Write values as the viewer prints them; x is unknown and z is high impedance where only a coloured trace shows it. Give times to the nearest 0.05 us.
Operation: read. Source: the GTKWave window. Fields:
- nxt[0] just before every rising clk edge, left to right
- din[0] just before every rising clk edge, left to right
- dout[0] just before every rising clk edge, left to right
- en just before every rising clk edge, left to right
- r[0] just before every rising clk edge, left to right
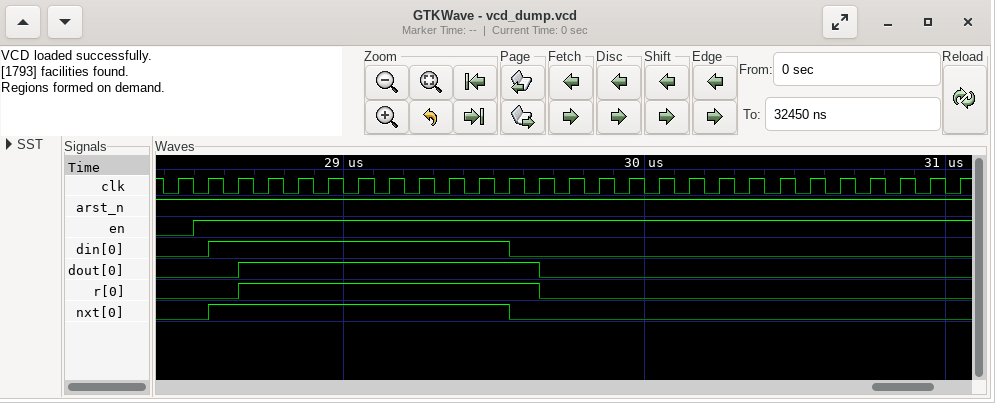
0 0 1 1 1 1 1 1 1 1 1 1 0 0 0 0 0 0 0 0 0 0 0 0 0 0 0
0 0 1 1 1 1 1 1 1 1 1 1 0 0 0 0 0 0 0 0 0 0 0 0 0 0 0
0 0 0 1 1 1 1 1 1 1 1 1 1 0 0 0 0 0 0 0 0 0 0 0 0 0 0
0 1 1 1 1 1 1 1 1 1 1 1 1 1 1 1 1 1 1 1 1 1 1 1 1 1 1
0 0 0 1 1 1 1 1 1 1 1 1 1 0 0 0 0 0 0 0 0 0 0 0 0 0 0
